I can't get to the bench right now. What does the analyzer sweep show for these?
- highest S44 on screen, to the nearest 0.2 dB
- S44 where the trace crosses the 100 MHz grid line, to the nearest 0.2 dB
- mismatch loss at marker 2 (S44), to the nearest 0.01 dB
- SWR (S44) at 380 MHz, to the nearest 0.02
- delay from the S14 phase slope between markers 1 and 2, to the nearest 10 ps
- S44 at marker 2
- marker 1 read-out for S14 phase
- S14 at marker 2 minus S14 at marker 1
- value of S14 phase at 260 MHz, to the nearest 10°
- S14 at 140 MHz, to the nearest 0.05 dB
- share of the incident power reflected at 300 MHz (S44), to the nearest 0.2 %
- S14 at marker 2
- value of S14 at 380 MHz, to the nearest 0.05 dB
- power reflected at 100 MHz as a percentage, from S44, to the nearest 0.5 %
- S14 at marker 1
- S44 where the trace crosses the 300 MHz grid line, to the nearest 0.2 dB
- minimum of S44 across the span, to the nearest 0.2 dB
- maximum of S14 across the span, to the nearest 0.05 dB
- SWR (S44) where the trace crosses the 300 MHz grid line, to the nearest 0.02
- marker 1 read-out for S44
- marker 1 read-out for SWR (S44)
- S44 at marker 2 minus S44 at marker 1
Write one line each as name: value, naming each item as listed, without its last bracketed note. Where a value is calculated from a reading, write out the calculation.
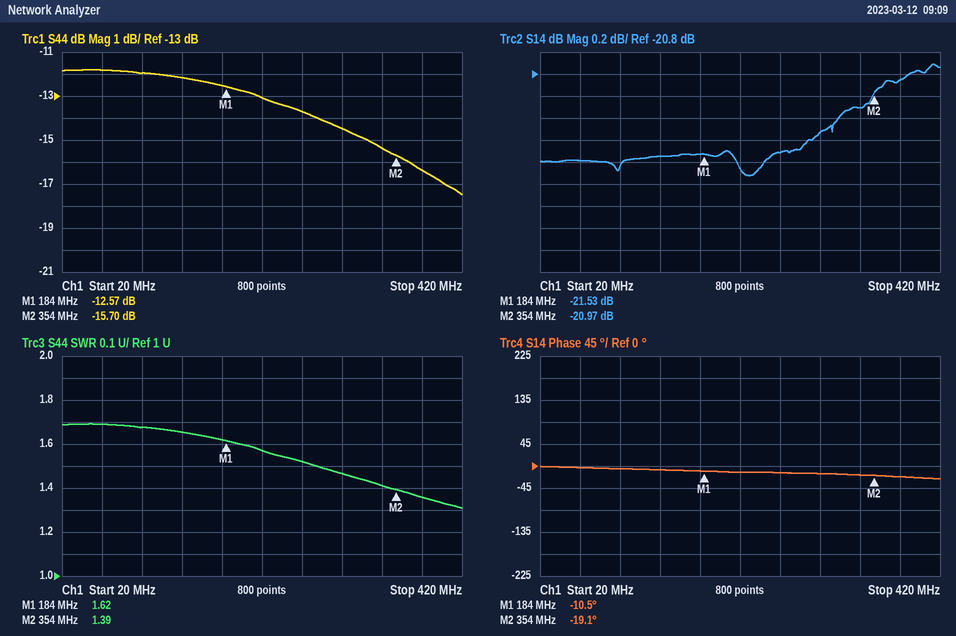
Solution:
highest S44 on screen, to the nearest 0.2 dB: -11.8 dB
S44 where the trace crosses the 100 MHz grid line, to the nearest 0.2 dB: -12.0 dB
mismatch loss at marker 2 (S44), to the nearest 0.01 dB: −10 log10(1 − 10^(-15.7/10)) ≈ 0.12 dB
SWR (S44) at 380 MHz, to the nearest 0.02: 1.36
delay from the S14 phase slope between markers 1 and 2, to the nearest 10 ps: −(-19.1° − (-10.5°))/(360° × 170 MHz) ≈ 141 ps, so 140 ps to the nearest 10 ps
S44 at marker 2: -15.70 dB
marker 1 read-out for S14 phase: -10.5°
S14 at marker 2 minus S14 at marker 1: -20.97 − (-21.53) = 0.56 dB
value of S14 phase at 260 MHz, to the nearest 10°: -10°
S14 at 140 MHz, to the nearest 0.05 dB: -21.55 dB
share of the incident power reflected at 300 MHz (S44), to the nearest 0.2 %: 10^(-14.4/10) ≈ 3.6 %
S14 at marker 2: -20.97 dB
value of S14 at 380 MHz, to the nearest 0.05 dB: -20.85 dB
power reflected at 100 MHz as a percentage, from S44, to the nearest 0.5 %: 10^(-12/10) ≈ 6.31 %, so 6.5 % to the nearest 0.5 %
S14 at marker 1: -21.53 dB
S44 where the trace crosses the 300 MHz grid line, to the nearest 0.2 dB: -14.4 dB
minimum of S44 across the span, to the nearest 0.2 dB: -17.4 dB
maximum of S14 across the span, to the nearest 0.05 dB: -20.70 dB
SWR (S44) where the trace crosses the 300 MHz grid line, to the nearest 0.02: 1.46
marker 1 read-out for S44: -12.57 dB
marker 1 read-out for SWR: 1.62
S44 at marker 2 minus S44 at marker 1: -15.7 − (-12.57) = -3.13 dB
